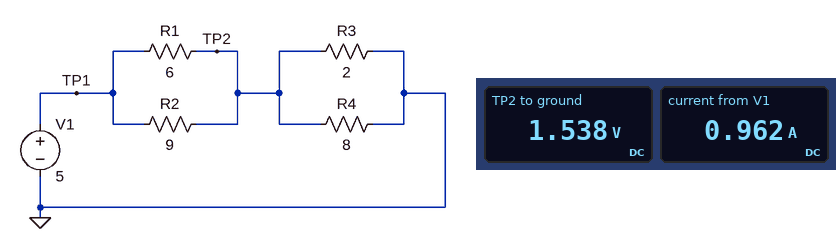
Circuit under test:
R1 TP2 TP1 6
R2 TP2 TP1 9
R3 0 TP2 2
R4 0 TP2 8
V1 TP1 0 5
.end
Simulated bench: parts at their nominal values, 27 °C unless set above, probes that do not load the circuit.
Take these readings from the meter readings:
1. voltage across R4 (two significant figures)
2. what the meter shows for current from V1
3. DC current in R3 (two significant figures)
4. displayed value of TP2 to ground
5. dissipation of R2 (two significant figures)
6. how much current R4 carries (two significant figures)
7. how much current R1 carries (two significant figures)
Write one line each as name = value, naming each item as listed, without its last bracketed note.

voltage across R4 = 1.5 V
what the meter shows for current from V1 = 0.962 A
DC current in R3 = 770 mA
displayed value of TP2 to ground = 1.538 V
dissipation of R2 = 1.3 W
how much current R4 carries = 190 mA
how much current R1 carries = 580 mA
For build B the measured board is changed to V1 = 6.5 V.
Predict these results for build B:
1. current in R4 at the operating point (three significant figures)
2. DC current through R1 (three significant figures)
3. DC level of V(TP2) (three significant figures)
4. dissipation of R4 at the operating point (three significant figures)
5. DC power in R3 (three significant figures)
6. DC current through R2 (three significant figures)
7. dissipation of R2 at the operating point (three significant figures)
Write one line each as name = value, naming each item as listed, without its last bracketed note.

current in R4 at the operating point = 250 mA
DC current through R1 = 750 mA
DC level of V(TP2) = 2.00 V
dissipation of R4 at the operating point = 500 mW
DC power in R3 = 2.00 W
DC current through R2 = 500 mA
dissipation of R2 at the operating point = 2.25 W
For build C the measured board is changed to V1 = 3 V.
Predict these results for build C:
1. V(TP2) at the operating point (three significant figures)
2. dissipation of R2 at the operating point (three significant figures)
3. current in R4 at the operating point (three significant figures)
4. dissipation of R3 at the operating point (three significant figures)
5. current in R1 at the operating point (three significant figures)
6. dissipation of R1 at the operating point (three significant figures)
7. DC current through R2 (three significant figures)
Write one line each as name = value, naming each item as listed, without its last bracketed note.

V(TP2) at the operating point = 923 mV
dissipation of R2 at the operating point = 479 mW
current in R4 at the operating point = 115 mA
dissipation of R3 at the operating point = 426 mW
current in R1 at the operating point = 346 mA
dissipation of R1 at the operating point = 719 mW
DC current through R2 = 231 mA
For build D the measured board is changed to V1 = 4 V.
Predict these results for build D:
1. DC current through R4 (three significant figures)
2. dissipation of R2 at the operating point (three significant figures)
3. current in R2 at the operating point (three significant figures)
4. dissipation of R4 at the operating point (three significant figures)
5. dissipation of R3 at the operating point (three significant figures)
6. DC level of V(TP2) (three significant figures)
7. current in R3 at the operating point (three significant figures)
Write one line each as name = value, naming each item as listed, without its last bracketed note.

DC current through R4 = 154 mA
dissipation of R2 at the operating point = 852 mW
current in R2 at the operating point = 308 mA
dissipation of R4 at the operating point = 189 mW
dissipation of R3 at the operating point = 757 mW
DC level of V(TP2) = 1.23 V
current in R3 at the operating point = 615 mA
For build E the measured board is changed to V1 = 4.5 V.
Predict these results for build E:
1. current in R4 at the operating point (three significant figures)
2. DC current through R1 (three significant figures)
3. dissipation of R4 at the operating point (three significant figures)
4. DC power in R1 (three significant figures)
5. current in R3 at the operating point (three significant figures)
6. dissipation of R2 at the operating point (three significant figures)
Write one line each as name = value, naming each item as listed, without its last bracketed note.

current in R4 at the operating point = 173 mA
DC current through R1 = 519 mA
dissipation of R4 at the operating point = 240 mW
DC power in R1 = 1.62 W
current in R3 at the operating point = 692 mA
dissipation of R2 at the operating point = 1.08 W
